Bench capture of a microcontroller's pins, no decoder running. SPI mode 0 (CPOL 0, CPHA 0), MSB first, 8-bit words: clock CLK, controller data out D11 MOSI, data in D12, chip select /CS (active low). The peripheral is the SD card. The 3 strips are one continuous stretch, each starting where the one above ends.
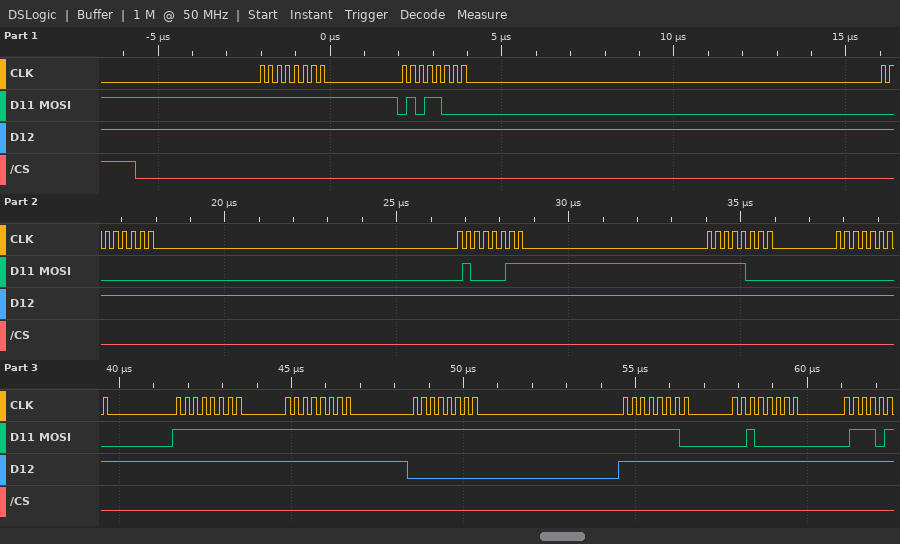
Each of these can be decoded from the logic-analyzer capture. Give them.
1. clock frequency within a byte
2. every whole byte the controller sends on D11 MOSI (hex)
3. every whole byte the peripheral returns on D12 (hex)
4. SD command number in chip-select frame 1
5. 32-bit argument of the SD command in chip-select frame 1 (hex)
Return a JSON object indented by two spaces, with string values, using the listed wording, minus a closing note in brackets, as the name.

{
  "clock frequency within a byte": "4 MHz",
  "every whole byte the controller sends on D11 MOSI": "FF 58 00 43 F8 00 FF FF FF FE 20",
  "every whole byte the peripheral returns on D12": "FF FF FF FF FF FF FF FF 00 FF FF",
  "SD command number in chip-select frame 1": "CMD24",
  "32-bit argument of the SD command in chip-select frame 1": "0x0043F800"
}
